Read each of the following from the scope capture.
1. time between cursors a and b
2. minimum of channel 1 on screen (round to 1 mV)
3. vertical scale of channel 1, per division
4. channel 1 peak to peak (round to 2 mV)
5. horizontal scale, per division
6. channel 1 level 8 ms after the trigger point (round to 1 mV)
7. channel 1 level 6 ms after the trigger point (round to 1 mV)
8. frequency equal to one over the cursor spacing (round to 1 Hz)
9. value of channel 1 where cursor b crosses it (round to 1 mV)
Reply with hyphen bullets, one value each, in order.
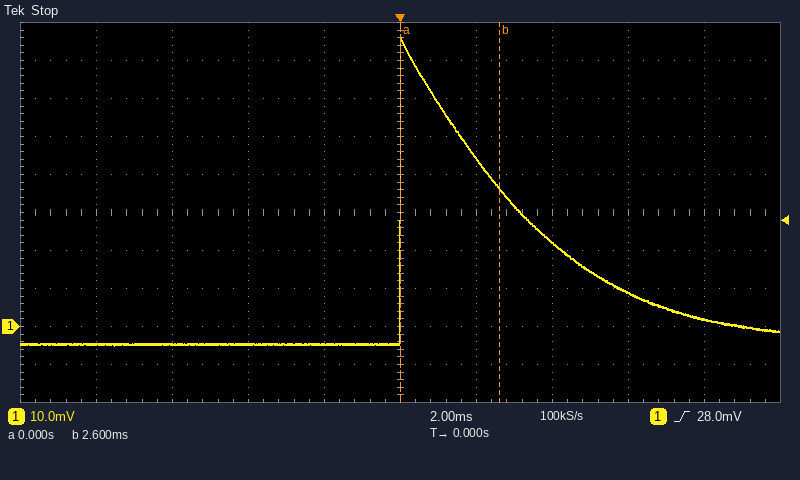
- 2.6 ms
- -5 mV
- 10 mV
- 82 mV
- 2 ms
- 2 mV
- 9 mV
- 385 Hz
- 36 mV
